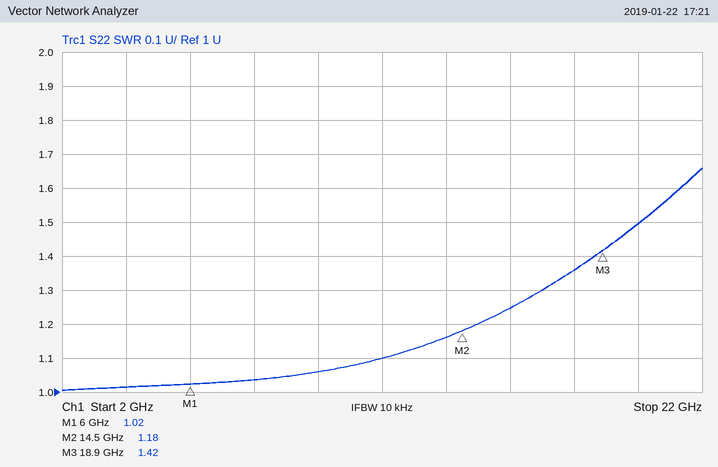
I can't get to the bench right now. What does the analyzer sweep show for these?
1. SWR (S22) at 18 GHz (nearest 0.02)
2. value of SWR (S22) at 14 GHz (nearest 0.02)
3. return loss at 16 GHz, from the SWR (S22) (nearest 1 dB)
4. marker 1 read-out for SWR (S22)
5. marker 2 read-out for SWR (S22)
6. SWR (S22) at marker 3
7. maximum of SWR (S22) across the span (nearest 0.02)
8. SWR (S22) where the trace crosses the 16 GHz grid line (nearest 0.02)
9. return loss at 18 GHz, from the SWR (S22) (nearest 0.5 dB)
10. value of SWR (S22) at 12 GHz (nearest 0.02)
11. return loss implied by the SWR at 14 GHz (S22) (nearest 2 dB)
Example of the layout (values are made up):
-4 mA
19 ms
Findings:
1.36
1.16
19 dB
1.02
1.18
1.42
1.66
1.24
16.5 dB
1.10
22 dB
